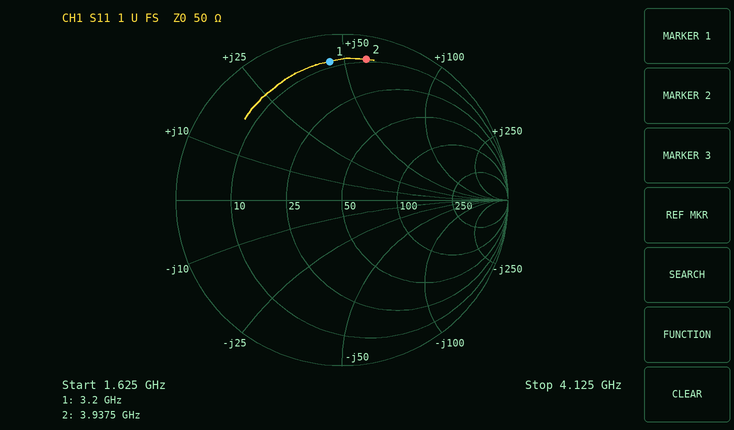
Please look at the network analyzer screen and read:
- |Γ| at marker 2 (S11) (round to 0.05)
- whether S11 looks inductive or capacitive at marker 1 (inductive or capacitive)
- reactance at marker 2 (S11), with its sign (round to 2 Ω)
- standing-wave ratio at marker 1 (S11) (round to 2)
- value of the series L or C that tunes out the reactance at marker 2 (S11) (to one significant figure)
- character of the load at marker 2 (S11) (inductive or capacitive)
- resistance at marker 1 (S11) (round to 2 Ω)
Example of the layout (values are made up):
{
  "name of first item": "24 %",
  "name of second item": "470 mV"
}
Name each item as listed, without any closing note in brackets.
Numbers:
{
  "|Γ| at marker 2 (S11)": "0.85",
  "whether S11 looks inductive or capacitive at marker 1": "inductive",
  "reactance at marker 2 (S11), with its sign": "+58 Ω",
  "standing-wave ratio at marker 1 (S11)": "12",
  "value of the series L or C that tunes out the reactance at marker 2 (S11)": "700 fF",
  "character of the load at marker 2 (S11)": "inductive",
  "resistance at marker 1 (S11)": "8 Ω"
}
